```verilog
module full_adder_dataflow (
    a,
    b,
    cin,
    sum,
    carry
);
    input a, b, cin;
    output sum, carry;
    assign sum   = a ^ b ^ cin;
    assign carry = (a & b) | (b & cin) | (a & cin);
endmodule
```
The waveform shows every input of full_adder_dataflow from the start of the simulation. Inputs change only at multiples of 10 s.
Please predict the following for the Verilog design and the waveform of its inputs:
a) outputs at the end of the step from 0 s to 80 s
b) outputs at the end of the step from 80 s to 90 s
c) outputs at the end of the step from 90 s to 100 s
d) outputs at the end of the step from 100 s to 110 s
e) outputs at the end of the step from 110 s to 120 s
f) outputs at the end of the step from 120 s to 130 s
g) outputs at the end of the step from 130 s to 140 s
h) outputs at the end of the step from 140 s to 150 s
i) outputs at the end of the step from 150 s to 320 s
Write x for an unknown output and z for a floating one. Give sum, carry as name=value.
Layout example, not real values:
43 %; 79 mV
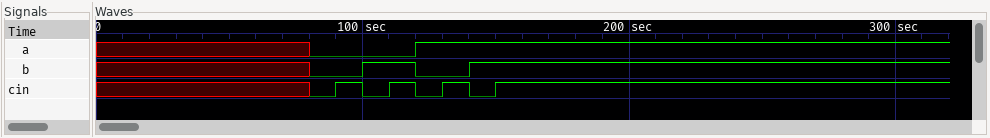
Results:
sum=x, carry=x; sum=0, carry=0; sum=1, carry=0; sum=1, carry=0; sum=0, carry=1; sum=1, carry=0; sum=0, carry=1; sum=0, carry=1; sum=1, carry=1
